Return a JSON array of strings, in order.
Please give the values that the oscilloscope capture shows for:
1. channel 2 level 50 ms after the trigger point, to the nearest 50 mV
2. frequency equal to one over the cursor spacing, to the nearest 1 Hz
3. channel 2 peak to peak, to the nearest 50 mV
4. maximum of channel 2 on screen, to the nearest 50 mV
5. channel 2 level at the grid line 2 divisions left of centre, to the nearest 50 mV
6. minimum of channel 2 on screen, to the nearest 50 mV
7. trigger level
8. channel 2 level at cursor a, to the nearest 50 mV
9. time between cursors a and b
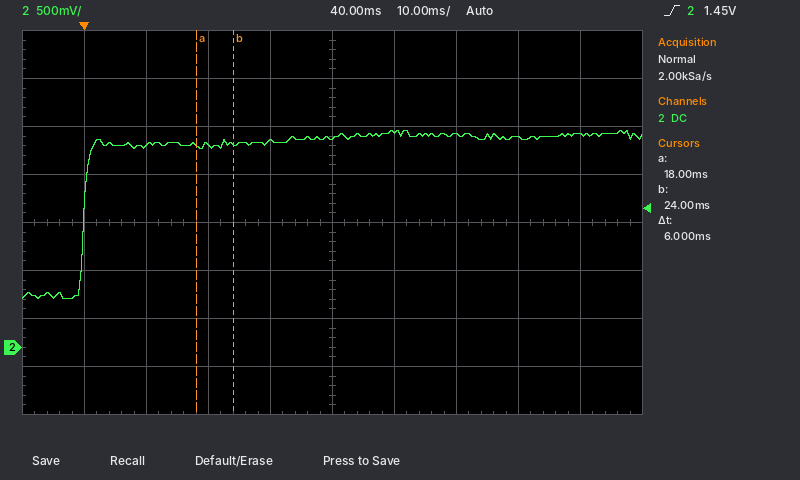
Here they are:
["2.25 V", "167 Hz", "1.75 V", "2.25 V", "2.10 V", "500 mV", "1.45 V", "2.10 V", "6 ms"]
